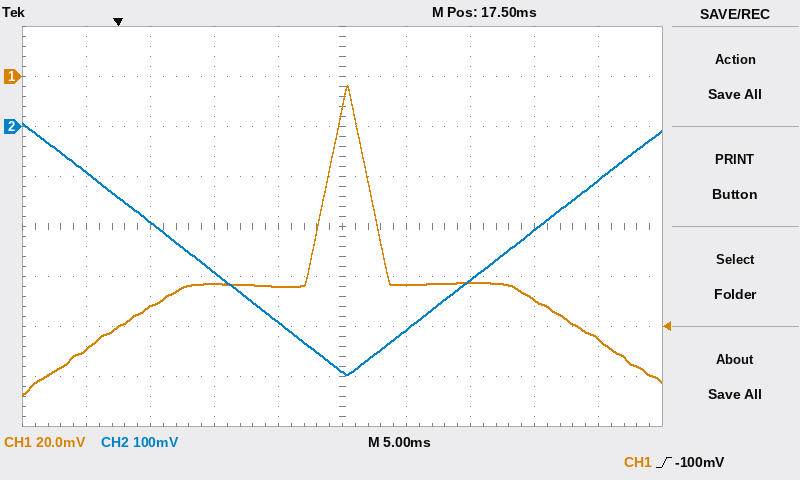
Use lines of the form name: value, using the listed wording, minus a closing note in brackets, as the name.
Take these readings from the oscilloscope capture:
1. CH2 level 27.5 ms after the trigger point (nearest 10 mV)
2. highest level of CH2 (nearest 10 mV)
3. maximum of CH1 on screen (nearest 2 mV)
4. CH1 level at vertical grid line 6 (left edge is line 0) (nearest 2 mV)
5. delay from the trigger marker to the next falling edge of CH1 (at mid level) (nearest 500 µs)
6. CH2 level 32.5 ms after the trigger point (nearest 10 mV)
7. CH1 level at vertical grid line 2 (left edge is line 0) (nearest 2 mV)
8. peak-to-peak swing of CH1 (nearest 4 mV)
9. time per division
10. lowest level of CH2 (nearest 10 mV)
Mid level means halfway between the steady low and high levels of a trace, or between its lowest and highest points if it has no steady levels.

CH2 level 27.5 ms after the trigger point: -310 mV
highest level of CH2: 10 mV
maximum of CH1 on screen: -4 mV
CH1 level at vertical grid line 6 (left edge is line 0): -84 mV
delay from the trigger marker to the next falling edge of CH1 (at mid level): 20.5 ms
CH2 level 32.5 ms after the trigger point: -210 mV
CH1 level at vertical grid line 2 (left edge is line 0): -92 mV
peak-to-peak swing of CH1: 124 mV
time per division: 5 ms
lowest level of CH2: -500 mV
